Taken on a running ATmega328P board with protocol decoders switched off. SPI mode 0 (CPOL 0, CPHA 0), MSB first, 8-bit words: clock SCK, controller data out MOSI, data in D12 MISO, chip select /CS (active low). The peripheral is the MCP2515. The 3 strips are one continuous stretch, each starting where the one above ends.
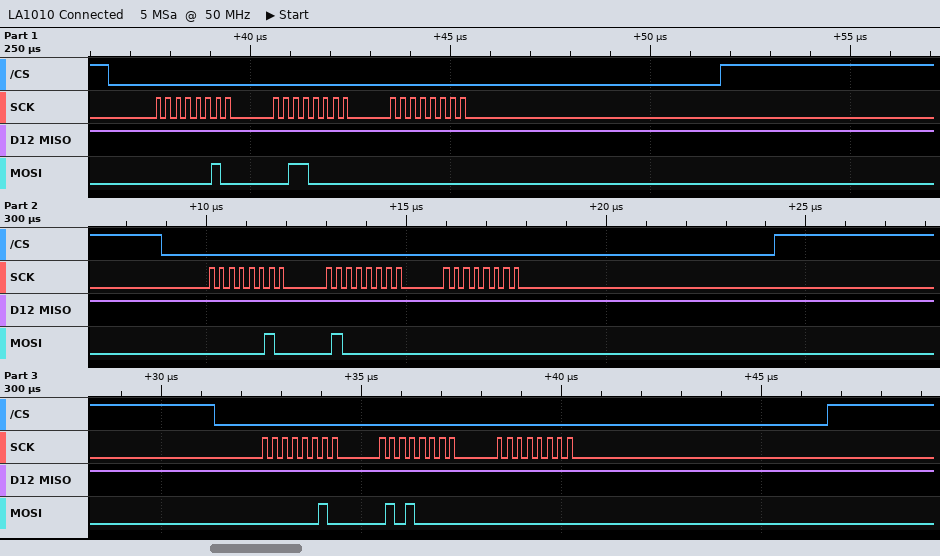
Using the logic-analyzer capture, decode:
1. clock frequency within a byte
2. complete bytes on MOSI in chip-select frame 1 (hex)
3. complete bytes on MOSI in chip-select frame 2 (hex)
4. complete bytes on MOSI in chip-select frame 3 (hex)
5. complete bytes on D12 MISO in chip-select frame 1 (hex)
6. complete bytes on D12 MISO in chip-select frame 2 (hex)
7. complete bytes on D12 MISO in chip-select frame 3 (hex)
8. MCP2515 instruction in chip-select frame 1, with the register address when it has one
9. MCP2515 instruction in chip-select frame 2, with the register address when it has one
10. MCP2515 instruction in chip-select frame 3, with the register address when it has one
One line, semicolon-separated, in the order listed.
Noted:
4 MHz; 02 30 00; 02 40 00; 02 50 00; FF FF FF; FF FF FF; FF FF FF; WRITE 0x30; WRITE 0x40; WRITE 0x50
